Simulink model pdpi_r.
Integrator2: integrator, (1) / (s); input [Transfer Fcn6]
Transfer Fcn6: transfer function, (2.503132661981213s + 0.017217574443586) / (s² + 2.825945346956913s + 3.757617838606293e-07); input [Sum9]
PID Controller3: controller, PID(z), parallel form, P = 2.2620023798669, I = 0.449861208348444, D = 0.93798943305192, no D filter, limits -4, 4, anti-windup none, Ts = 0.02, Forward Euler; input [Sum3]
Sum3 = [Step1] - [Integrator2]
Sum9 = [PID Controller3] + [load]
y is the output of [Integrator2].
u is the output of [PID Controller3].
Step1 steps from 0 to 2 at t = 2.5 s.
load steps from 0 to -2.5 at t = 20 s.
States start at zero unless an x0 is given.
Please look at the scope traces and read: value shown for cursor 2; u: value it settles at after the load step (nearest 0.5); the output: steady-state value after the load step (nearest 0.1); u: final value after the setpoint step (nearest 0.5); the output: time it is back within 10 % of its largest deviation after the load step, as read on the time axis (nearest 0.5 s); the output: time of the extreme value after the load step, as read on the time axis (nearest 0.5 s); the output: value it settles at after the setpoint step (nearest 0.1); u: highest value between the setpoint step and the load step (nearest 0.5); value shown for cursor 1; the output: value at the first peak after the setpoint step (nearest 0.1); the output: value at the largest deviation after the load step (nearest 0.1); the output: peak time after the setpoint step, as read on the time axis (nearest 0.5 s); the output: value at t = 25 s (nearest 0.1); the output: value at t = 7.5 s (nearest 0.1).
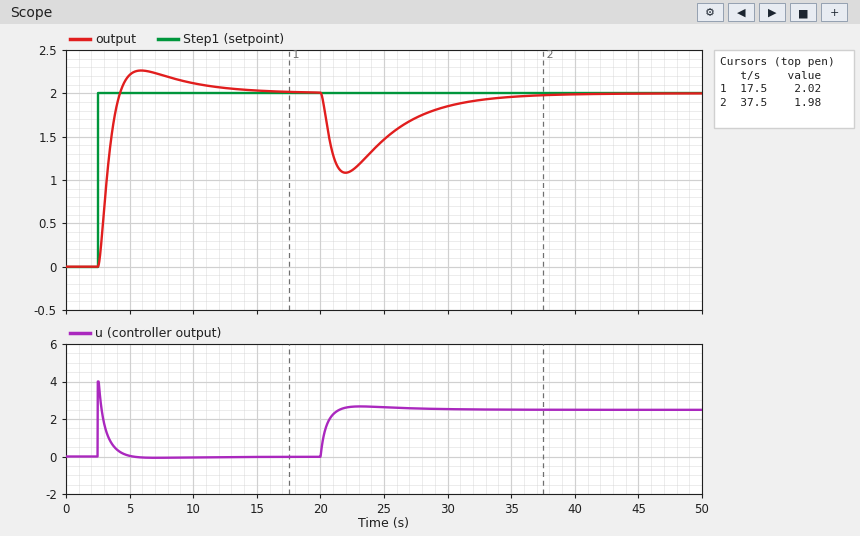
1.98
2.5
2.0
0.0
32.0 s
22.0 s
2.0
4.0
2.02
2.3
1.1
6.0 s
1.5
2.2
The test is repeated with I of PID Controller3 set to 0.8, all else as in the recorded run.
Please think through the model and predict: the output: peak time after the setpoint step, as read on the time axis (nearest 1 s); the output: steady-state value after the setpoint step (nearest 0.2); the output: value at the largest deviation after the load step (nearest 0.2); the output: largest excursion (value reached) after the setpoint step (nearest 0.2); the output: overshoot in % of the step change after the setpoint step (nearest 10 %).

5 s
2.0
1.2
2.4
20 %
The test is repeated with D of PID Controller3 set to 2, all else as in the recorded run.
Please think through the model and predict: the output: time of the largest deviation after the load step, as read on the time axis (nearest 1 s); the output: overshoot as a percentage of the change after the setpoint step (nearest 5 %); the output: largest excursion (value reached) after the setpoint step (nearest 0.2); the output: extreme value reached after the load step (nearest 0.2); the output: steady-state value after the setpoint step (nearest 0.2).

23 s
15 %
2.4
1.2
2.0
